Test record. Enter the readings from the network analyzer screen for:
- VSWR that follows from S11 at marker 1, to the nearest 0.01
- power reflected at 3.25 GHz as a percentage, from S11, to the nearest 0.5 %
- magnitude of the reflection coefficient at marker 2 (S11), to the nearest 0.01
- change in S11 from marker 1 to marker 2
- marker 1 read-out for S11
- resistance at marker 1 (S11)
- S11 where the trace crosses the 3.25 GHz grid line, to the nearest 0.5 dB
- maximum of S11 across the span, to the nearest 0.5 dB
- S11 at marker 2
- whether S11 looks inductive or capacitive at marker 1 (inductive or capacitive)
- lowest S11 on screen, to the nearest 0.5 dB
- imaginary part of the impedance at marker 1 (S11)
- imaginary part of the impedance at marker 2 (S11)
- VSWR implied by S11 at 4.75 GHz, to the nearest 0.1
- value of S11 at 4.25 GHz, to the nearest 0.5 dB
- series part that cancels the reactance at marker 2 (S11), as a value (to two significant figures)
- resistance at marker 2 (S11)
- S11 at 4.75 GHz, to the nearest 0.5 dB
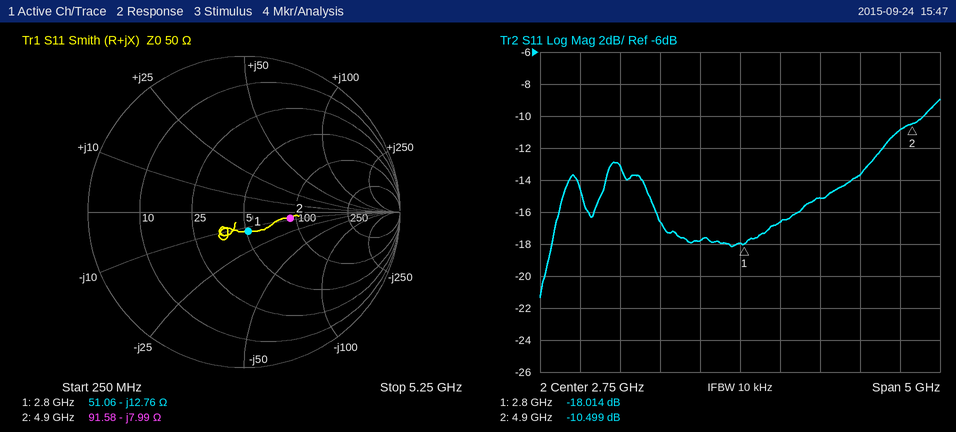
1.29
2.0 %
0.30
7.515 dB
-18.014 dB
51.06 Ω
-16.5 dB
-9.0 dB
-10.499 dB
capacitive
-21.5 dB
-12.76 Ω
-7.99 Ω
1.8
-13.5 dB
260 pH
91.58 Ω
-11.0 dB
